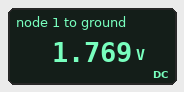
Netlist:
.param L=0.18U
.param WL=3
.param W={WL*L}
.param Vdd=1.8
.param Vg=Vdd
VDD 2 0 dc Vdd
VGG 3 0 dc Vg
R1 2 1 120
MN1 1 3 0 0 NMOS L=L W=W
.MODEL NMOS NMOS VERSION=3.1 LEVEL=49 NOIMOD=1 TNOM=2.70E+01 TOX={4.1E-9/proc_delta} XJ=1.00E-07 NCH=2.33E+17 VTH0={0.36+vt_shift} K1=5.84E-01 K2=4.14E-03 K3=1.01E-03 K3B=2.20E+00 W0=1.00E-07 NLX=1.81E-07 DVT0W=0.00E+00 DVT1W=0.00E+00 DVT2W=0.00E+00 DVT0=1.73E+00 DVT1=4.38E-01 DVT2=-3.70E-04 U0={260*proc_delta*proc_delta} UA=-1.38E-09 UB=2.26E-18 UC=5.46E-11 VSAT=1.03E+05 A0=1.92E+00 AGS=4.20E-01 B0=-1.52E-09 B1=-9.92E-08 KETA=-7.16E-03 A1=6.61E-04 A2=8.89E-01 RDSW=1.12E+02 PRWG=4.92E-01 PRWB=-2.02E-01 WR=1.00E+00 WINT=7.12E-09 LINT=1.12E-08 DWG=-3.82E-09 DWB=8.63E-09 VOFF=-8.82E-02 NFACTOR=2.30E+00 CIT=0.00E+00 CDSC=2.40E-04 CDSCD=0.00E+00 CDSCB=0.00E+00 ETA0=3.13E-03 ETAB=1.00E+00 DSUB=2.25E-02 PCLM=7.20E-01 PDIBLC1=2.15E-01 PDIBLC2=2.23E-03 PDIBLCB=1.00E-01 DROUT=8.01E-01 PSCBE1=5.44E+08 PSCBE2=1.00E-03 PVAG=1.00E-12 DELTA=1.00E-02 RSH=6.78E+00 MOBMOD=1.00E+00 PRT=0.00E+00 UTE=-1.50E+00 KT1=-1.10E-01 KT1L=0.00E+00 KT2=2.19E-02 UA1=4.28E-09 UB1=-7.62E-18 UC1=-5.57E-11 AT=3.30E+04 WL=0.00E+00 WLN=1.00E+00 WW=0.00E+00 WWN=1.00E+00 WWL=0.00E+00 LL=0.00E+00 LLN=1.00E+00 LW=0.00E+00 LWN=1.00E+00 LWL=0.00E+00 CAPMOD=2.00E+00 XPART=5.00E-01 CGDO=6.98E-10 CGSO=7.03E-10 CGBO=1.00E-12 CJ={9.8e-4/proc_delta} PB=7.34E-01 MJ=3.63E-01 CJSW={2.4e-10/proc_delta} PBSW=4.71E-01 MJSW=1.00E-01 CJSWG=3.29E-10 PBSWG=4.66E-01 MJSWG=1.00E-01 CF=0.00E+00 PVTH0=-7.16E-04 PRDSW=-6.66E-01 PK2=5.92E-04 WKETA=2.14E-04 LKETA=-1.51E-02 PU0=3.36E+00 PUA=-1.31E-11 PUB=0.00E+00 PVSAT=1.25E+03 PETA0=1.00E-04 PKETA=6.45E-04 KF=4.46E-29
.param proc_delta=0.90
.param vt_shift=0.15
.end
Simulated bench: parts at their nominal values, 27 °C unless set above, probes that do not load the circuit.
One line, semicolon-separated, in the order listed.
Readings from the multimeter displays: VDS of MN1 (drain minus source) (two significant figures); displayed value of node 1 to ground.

1.8 V; 1.769 V
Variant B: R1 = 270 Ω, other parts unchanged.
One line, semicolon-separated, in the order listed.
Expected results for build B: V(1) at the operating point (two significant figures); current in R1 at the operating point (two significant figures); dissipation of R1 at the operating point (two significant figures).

1.7 V; 260 µA; 18 µW
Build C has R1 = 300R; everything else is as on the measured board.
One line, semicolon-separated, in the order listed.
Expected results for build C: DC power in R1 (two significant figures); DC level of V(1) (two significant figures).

20 µW; 1.7 V
